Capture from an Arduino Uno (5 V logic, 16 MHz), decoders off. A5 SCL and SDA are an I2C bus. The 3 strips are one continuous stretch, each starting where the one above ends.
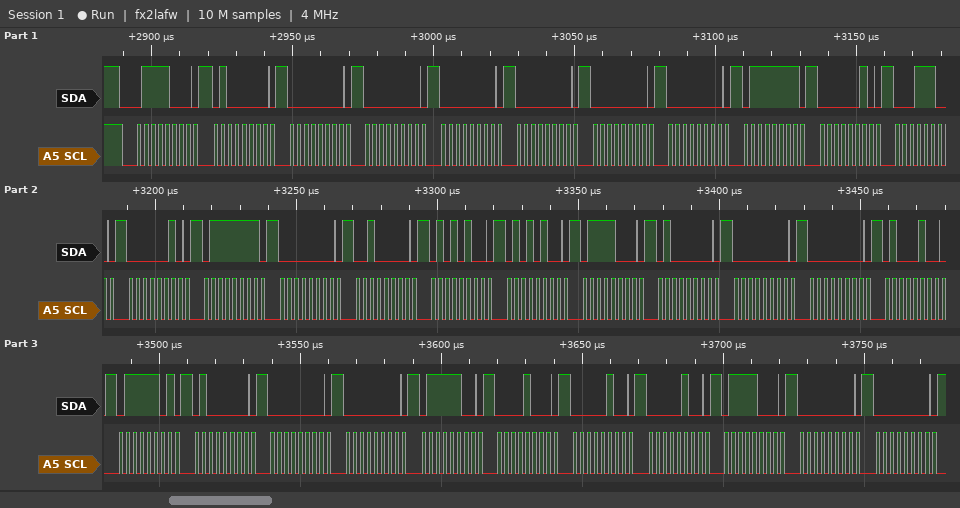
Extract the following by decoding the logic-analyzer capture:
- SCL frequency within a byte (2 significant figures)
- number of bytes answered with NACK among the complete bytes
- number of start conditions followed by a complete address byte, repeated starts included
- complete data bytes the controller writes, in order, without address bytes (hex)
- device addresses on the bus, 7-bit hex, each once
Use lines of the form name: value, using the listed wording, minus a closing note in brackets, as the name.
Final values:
SCL frequency within a byte: 400 kHz
number of bytes answered with NACK among the complete bytes: 0
number of start conditions followed by a complete address byte, repeated starts included: 1
complete data bytes the controller writes, in order, without address bytes: 40 00 00 00 00 00 00 7F 02 1C 02 7F 00 20 54 54 78 40 00 00 44 7D 40 00 00 7C 08 04 04 78 00 00
device addresses on the bus, 7-bit hex, each once: 0x3C
